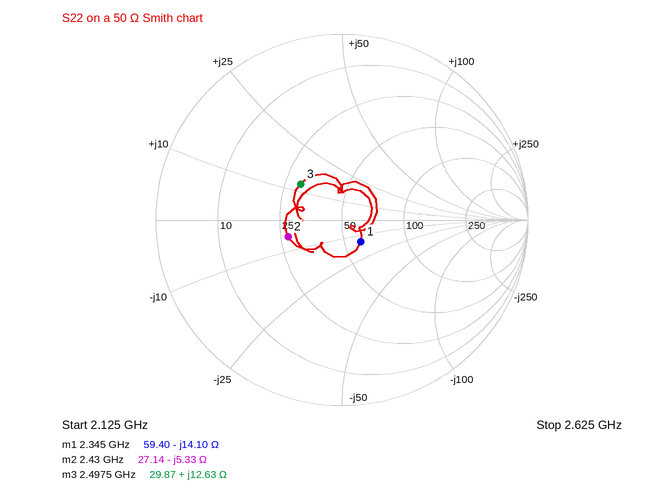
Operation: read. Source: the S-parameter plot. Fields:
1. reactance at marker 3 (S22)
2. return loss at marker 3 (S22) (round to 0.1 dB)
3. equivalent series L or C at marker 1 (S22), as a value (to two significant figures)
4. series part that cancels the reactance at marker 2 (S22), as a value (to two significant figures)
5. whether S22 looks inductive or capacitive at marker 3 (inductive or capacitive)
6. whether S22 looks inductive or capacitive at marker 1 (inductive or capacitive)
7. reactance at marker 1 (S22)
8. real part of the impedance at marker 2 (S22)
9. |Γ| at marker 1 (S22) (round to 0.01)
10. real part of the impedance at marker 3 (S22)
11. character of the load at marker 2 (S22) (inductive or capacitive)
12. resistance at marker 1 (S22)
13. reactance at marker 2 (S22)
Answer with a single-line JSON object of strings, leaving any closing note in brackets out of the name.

{"reactance at marker 3": "+12.63 Ω", "return loss at marker 3 (S22)": "10.6 dB", "equivalent series L or C at marker 1 (S22), as a value": "4.8 pF", "series part that cancels the reactance at marker 2 (S22), as a value": "350 pH", "whether S22 looks inductive or capacitive at marker 3": "inductive", "whether S22 looks inductive or capacitive at marker 1": "capacitive", "reactance at marker 1": "-14.10 Ω", "real part of the impedance at marker 2": "27.14 Ω", "|Γ| at marker 1 (S22)": "0.15", "real part of the impedance at marker 3": "29.87 Ω", "character of the load at marker 2 (S22)": "capacitive", "resistance at marker 1": "59.40 Ω", "reactance at marker 2": "-5.33 Ω"}
